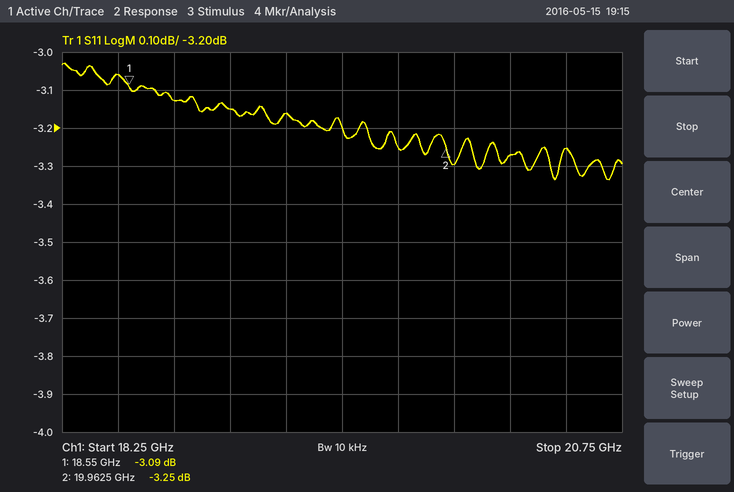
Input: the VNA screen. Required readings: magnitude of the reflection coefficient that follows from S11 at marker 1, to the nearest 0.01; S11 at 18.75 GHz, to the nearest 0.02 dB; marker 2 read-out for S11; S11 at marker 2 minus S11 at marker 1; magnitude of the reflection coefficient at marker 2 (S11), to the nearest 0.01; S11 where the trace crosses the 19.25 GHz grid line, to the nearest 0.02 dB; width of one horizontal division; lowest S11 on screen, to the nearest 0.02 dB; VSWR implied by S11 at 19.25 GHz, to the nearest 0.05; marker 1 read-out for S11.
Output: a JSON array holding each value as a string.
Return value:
["0.70", "-3.12 dB", "-3.25 dB", "-0.16 dB", "0.69", "-3.16 dB", "250 MHz", "-3.34 dB", "5.55", "-3.09 dB"]
